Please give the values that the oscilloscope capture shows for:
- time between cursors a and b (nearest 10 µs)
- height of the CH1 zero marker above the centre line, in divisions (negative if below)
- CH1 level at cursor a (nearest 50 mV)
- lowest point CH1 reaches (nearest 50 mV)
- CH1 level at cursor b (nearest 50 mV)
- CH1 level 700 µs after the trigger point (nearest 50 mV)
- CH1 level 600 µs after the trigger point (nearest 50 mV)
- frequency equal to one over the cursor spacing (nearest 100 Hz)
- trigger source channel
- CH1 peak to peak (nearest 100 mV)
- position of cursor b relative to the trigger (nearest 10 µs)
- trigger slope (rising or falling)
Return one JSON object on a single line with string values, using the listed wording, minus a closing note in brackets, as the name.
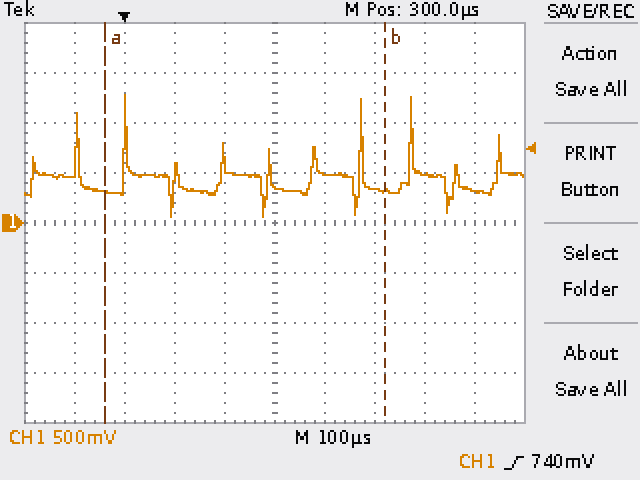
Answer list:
{"time between cursors a and b": "560 µs", "height of the CH1 zero marker above the centre line, in divisions": "0.0 div", "CH1 level at cursor a": "300 mV", "lowest point CH1 reaches": "50 mV", "CH1 level at cursor b": "300 mV", "CH1 level 700 µs after the trigger point": "300 mV", "CH1 level 600 µs after the trigger point": "500 mV", "frequency equal to one over the cursor spacing": "1.8 kHz", "trigger source channel": "CH1", "CH1 peak to peak": "1.20 V", "position of cursor b relative to the trigger": "+520 µs", "trigger slope": "rising"}
